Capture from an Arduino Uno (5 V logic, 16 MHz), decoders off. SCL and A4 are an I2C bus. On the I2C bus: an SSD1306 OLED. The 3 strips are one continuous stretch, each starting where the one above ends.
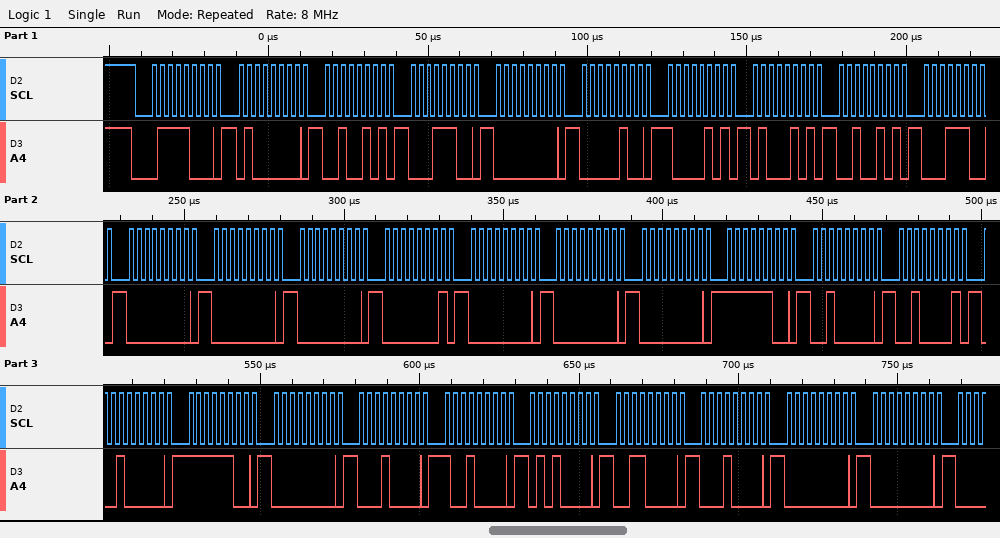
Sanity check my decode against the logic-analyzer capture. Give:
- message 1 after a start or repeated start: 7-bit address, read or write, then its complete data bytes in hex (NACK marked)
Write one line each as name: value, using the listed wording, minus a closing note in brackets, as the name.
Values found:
message 1 after a start or repeated start: 7-bit address, read or write, then its complete data bytes in hex: 0x3C write: 40 25 1C 00 04 85 45 25 1C 00 00 00 01 00 00 00 FC 20 21 20 FC 00 10 90 50 30 10 00 00
